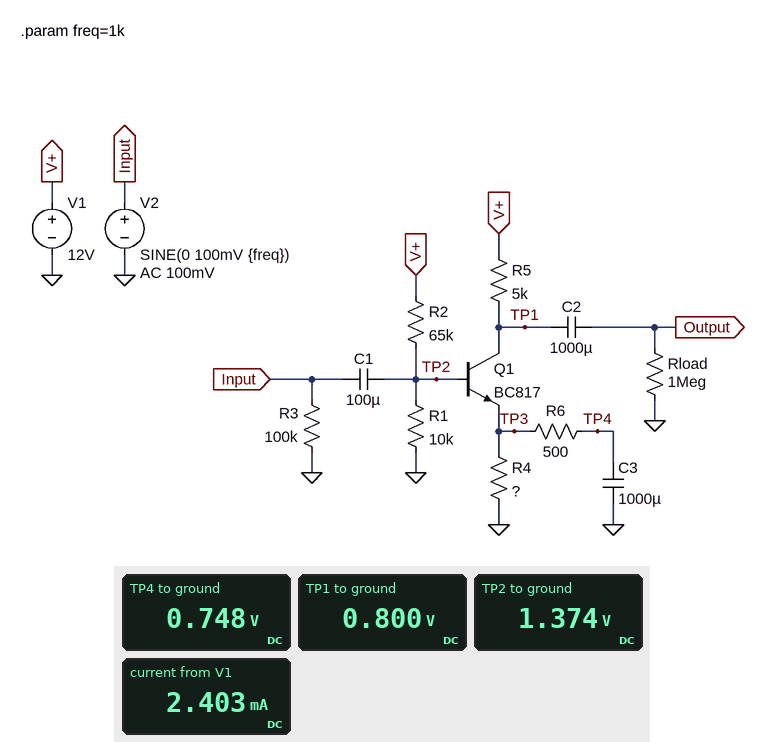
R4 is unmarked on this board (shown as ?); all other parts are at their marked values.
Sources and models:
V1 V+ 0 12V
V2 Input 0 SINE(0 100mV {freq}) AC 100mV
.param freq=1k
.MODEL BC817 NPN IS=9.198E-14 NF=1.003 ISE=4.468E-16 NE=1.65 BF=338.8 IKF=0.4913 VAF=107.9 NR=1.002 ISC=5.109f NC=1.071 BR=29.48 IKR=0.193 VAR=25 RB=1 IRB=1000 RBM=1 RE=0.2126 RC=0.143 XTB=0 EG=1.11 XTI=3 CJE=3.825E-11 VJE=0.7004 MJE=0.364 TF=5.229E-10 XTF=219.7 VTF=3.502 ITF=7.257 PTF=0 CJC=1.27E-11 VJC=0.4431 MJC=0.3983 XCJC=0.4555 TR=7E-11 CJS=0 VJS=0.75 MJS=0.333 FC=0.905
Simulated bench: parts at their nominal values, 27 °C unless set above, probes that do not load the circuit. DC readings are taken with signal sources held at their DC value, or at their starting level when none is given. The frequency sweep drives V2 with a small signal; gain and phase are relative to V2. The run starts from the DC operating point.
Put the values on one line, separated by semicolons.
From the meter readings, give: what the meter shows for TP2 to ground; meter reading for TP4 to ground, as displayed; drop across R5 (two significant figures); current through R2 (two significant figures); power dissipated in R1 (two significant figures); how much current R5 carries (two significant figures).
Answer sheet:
1.374 V; 0.748 V; 11 V; 160 µA; 190 µW; 2.2 mA
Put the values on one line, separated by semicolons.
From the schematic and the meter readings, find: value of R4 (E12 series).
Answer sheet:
330 Ω
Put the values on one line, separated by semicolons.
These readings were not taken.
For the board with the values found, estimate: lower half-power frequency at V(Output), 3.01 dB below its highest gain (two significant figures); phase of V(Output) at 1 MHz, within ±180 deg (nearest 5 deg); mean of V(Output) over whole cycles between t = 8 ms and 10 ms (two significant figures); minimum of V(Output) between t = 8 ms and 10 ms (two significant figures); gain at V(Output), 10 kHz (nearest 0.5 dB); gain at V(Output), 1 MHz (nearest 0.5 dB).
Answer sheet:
3.8 Hz; 145 deg; 740 mV; -15 mV; 6.5 dB; 6.0 dB
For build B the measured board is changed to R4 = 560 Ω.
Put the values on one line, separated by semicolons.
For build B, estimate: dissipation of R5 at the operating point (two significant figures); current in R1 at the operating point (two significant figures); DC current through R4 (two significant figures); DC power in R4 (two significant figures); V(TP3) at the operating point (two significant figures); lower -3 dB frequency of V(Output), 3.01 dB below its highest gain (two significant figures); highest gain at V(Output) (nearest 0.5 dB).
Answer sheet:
14 mW; 160 µA; 1.7 mA; 1.6 mW; 940 mV; 350 mHz; 25.0 dB
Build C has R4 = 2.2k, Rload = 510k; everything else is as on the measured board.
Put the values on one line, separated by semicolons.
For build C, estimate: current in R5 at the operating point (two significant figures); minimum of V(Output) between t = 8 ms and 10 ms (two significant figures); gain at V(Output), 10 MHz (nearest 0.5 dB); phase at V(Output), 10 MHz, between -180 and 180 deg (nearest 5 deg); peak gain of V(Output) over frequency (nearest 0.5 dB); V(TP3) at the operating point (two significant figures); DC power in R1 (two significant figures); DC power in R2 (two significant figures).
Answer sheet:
460 µA; -1.1 V; 16.5 dB; 110 deg; 20.5 dB; 1.0 V; 250 µW; 1.7 mW
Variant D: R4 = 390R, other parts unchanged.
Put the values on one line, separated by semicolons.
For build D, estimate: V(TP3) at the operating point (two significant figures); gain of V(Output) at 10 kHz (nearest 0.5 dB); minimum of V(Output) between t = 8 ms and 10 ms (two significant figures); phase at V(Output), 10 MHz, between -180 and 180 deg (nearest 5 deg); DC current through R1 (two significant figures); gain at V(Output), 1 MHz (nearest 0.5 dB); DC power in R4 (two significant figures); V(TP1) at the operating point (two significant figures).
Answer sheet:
870 mV; 15.5 dB; -38 mV; 40 deg; 150 µA; 13.5 dB; 1.9 mW; 950 mV
